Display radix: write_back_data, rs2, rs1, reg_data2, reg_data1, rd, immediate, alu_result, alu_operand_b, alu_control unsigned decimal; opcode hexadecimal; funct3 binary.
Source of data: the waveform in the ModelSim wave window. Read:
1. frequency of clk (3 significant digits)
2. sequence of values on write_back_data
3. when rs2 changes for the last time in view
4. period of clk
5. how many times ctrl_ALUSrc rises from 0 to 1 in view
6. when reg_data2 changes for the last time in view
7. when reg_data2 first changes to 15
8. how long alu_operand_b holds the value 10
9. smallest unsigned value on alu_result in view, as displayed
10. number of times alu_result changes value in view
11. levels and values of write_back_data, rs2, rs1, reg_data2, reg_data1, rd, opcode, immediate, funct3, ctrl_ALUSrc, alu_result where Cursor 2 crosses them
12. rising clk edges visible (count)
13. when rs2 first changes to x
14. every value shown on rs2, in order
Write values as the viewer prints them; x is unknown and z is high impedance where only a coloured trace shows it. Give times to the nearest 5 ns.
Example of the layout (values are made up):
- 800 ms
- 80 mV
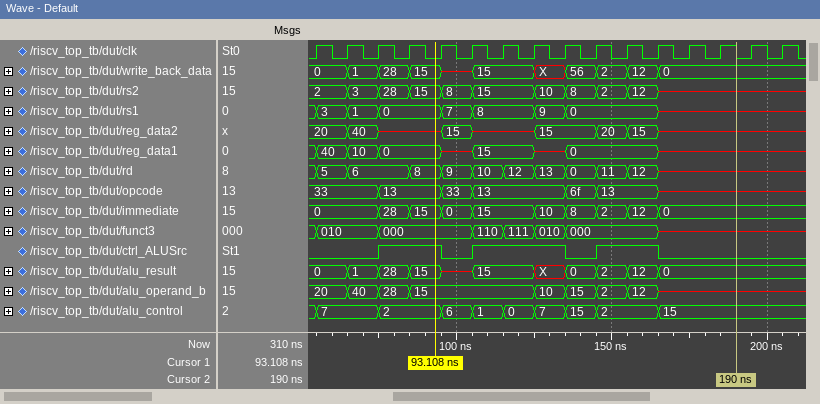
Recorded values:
- 100 MHz
- 0, 1, 28, 15, x, 15, X, 56, 2, 12, 0
- 165 ns
- 10 ns
- 3
- 165 ns
- 95 ns
- 10 ns
- 0
- 10
- write_back_data=0, rs2=x, rs1=x, reg_data2=x, reg_data1=x, rd=x, opcode=x, immediate=0, funct3=x, ctrl_ALUSrc=0, alu_result=0
- 16
- 165 ns
- 2, 3, 28, 15, 8, 15, 10, 8, 2, 12, x
